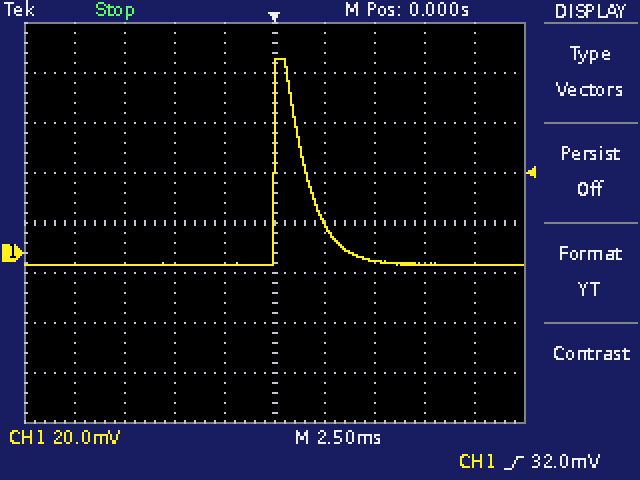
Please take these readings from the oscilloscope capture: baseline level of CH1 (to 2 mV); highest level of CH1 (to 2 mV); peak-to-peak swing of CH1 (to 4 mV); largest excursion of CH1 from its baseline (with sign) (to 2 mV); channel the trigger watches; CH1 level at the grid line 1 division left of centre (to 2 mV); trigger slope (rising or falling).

-4 mV
78 mV
84 mV
+82 mV
CH1
-4 mV
rising
